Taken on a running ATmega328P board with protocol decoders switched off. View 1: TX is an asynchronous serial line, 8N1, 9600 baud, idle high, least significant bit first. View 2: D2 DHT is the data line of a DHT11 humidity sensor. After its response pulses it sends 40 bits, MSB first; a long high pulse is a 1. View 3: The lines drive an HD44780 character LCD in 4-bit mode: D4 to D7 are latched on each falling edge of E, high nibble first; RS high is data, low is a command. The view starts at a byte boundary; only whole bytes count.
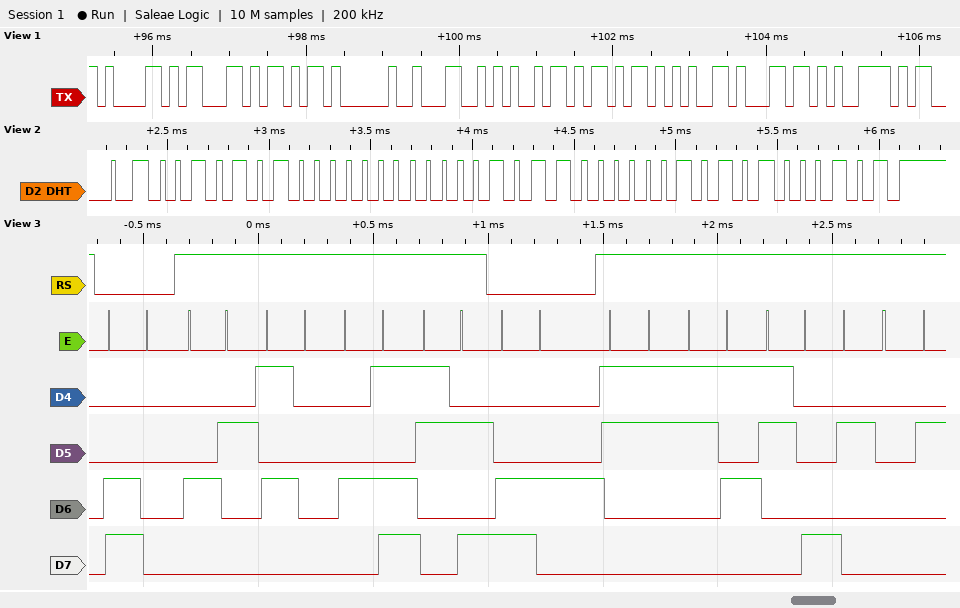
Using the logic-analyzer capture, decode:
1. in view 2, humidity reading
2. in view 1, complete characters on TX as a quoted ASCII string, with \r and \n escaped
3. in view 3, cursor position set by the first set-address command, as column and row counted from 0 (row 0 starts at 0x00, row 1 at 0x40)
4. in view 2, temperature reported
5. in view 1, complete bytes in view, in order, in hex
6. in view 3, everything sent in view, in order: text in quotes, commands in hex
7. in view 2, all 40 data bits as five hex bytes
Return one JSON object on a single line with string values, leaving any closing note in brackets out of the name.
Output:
{"in view 2, humidity reading": "42 %", "in view 1, complete characters on TX as a quoted ASCII string, with \\r and \\n escaped": "\"ack Likely\"", "in view 3, cursor position set by the first set-address command, as column and row counted from 0": "column 0, row 1", "in view 2, temperature reported": "22.5 °C", "in view 1, complete bytes in view, in order, in hex": "61 63 6B 20 4C 69 6B 65 6C 79", "in view 3, everything sent in view, in order: text in quotes, commands in hex": "0xC0 \"BPM:\" 0xC4 \"358 \"", "in view 2, all 40 data bits as five hex bytes": "2A 00 16 05 45"}
